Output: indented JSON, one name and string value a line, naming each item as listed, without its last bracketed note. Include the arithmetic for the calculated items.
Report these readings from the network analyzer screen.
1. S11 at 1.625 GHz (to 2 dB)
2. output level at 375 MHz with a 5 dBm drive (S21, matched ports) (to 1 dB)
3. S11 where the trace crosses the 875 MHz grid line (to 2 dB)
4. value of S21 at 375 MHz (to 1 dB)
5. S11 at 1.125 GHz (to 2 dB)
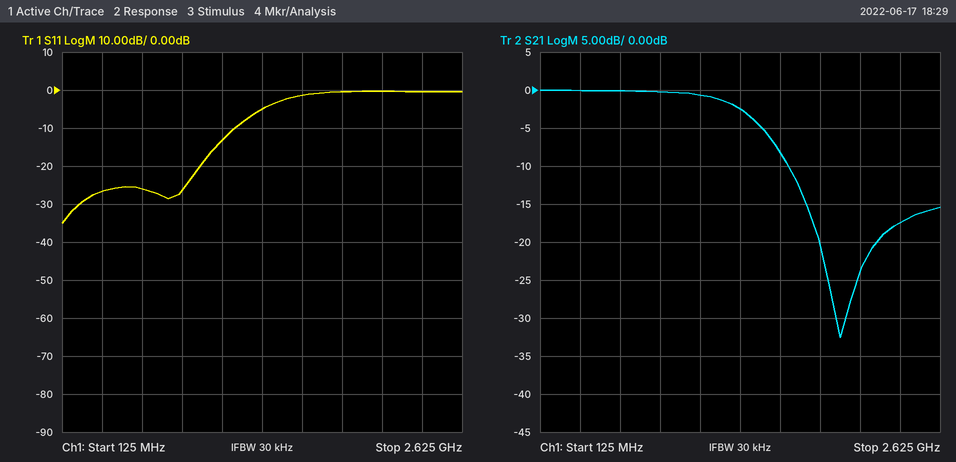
{
  "S11 at 1.625 GHz": "-2 dB",
  "output level at 375 MHz with a 5 dBm drive (S21, matched ports)": "5 dBm + (0 dB) = 5 dBm",
  "S11 where the trace crosses the 875 MHz grid line": "-26 dB",
  "value of S21 at 375 MHz": "0 dB",
  "S11 at 1.125 GHz": "-14 dB"
}
